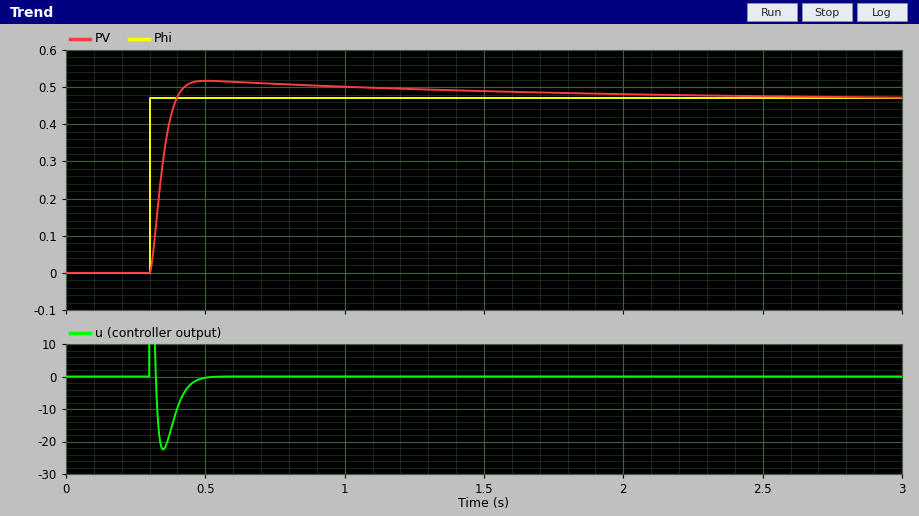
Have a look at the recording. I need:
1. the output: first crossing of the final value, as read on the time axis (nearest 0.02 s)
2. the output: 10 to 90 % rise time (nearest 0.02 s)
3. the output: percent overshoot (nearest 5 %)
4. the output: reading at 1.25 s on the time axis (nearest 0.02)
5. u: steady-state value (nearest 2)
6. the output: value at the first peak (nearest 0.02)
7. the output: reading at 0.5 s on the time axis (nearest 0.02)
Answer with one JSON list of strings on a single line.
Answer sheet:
["0.40 s", "0.06 s", "10 %", "0.50", "0", "0.52", "0.52"]
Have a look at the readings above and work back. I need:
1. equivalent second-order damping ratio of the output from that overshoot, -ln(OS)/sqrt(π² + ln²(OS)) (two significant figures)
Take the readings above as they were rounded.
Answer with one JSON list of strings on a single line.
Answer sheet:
["0.59"]
